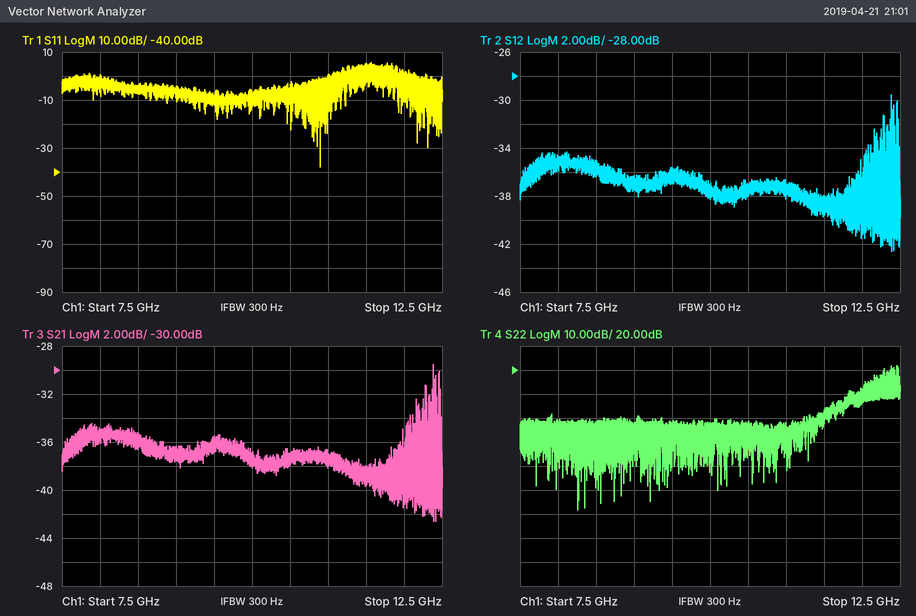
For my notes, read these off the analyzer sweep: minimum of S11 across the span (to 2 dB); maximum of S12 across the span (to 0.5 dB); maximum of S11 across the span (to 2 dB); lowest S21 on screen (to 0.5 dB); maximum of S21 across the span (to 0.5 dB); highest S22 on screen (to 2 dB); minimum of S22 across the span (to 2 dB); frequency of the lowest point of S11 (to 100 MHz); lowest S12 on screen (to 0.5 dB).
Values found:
-38 dB
-29.5 dB
6 dB
-42.5 dB
-29.5 dB
22 dB
-38 dB
10.9 GHz
-42.5 dB
